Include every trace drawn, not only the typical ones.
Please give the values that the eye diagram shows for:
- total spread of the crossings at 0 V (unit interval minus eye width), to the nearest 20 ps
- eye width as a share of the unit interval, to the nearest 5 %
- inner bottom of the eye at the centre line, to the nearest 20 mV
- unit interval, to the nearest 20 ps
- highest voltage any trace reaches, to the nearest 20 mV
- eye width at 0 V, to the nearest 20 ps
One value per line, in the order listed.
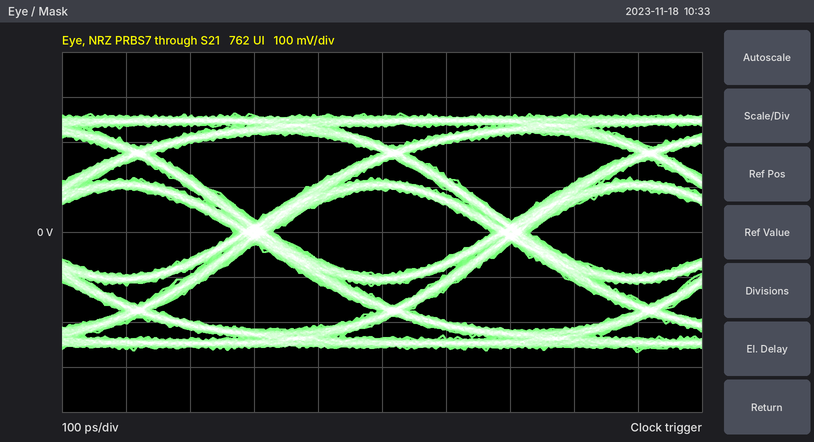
60 ps
85 %
-100 mV
400 ps
260 mV
340 ps
